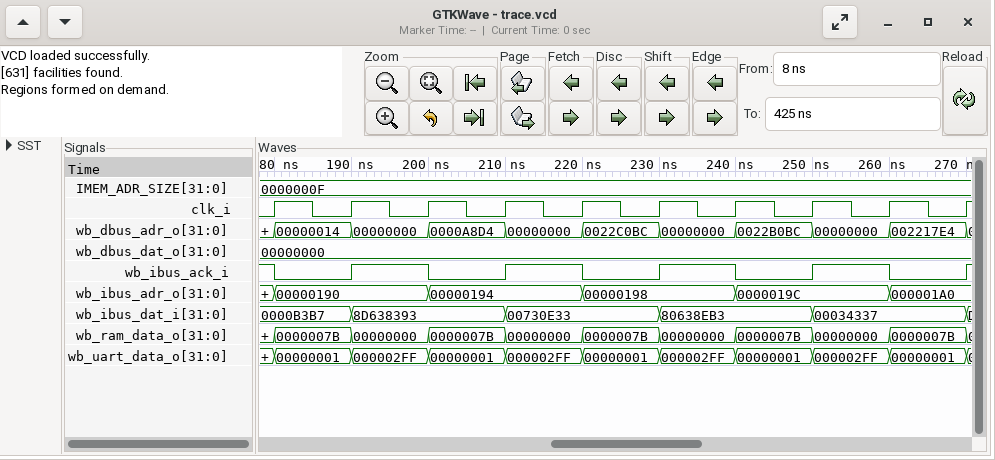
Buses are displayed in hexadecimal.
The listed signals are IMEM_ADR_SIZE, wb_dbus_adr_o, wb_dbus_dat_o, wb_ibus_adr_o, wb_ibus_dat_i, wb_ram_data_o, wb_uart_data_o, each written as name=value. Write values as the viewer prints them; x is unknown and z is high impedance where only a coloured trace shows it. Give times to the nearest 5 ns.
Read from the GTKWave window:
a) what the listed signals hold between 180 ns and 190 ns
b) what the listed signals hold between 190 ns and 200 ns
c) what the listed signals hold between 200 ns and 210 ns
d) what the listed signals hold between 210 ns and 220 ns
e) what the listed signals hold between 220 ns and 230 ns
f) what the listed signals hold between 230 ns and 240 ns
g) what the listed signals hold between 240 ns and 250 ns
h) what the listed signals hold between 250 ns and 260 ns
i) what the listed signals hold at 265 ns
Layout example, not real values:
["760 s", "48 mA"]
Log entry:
["IMEM_ADR_SIZE=0000000F, wb_dbus_adr_o=00000014, wb_dbus_dat_o=00000000, wb_ibus_adr_o=00000190, wb_ibus_dat_i=0000B3B7, wb_ram_data_o=0000007B, wb_uart_data_o=00000001", "IMEM_ADR_SIZE=0000000F, wb_dbus_adr_o=00000000, wb_dbus_dat_o=00000000, wb_ibus_adr_o=00000190, wb_ibus_dat_i=8D638393, wb_ram_data_o=00000000, wb_uart_data_o=000002FF", "IMEM_ADR_SIZE=0000000F, wb_dbus_adr_o=0000A8D4, wb_dbus_dat_o=00000000, wb_ibus_adr_o=00000194, wb_ibus_dat_i=8D638393, wb_ram_data_o=0000007B, wb_uart_data_o=00000001", "IMEM_ADR_SIZE=0000000F, wb_dbus_adr_o=00000000, wb_dbus_dat_o=00000000, wb_ibus_adr_o=00000194, wb_ibus_dat_i=00730E33, wb_ram_data_o=00000000, wb_uart_data_o=000002FF", "IMEM_ADR_SIZE=0000000F, wb_dbus_adr_o=0022C0BC, wb_dbus_dat_o=00000000, wb_ibus_adr_o=00000198, wb_ibus_dat_i=00730E33, wb_ram_data_o=0000007B, wb_uart_data_o=00000001", "IMEM_ADR_SIZE=0000000F, wb_dbus_adr_o=00000000, wb_dbus_dat_o=00000000, wb_ibus_adr_o=00000198, wb_ibus_dat_i=80638EB3, wb_ram_data_o=00000000, wb_uart_data_o=000002FF", "IMEM_ADR_SIZE=0000000F, wb_dbus_adr_o=0022B0BC, wb_dbus_dat_o=00000000, wb_ibus_adr_o=0000019C, wb_ibus_dat_i=80638EB3, wb_ram_data_o=0000007B, wb_uart_data_o=00000001", "IMEM_ADR_SIZE=0000000F, wb_dbus_adr_o=00000000, wb_dbus_dat_o=00000000, wb_ibus_adr_o=0000019C, wb_ibus_dat_i=00034337, wb_ram_data_o=00000000, wb_uart_data_o=000002FF", "IMEM_ADR_SIZE=0000000F, wb_dbus_adr_o=002217E4, wb_dbus_dat_o=00000000, wb_ibus_adr_o=000001A0, wb_ibus_dat_i=00034337, wb_ram_data_o=0000007B, wb_uart_data_o=00000001"]
